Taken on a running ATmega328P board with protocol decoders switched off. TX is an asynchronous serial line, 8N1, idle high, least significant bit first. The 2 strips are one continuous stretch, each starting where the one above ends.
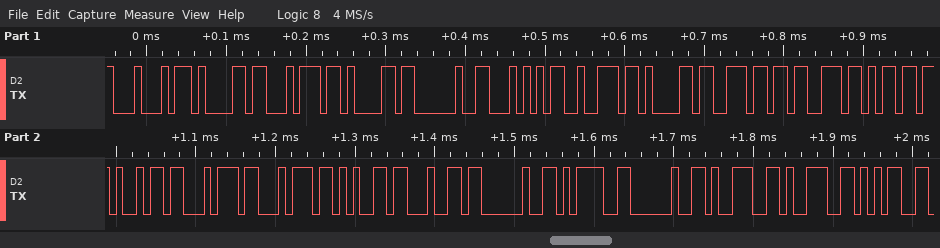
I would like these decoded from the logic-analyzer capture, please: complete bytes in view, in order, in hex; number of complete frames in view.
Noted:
44 61 74 61 20 54 72 61 6E 73 6D 69 74 74 65 64 20 3D 20 39 39 35
22
